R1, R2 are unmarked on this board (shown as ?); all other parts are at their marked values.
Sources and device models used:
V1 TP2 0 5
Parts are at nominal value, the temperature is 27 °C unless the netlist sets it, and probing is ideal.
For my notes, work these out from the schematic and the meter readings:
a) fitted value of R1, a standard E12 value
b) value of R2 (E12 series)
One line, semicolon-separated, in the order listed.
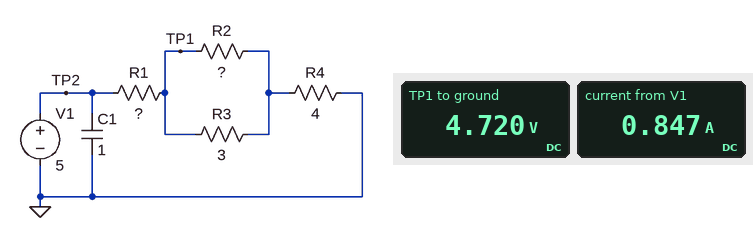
0.33 Ω; 3.3 Ω
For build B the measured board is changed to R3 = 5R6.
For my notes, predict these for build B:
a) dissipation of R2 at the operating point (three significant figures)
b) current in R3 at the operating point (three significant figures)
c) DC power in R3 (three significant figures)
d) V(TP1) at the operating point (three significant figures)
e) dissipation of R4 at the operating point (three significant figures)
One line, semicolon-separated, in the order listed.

796 mW; 289 mA; 469 mW; 4.74 V; 2.44 W
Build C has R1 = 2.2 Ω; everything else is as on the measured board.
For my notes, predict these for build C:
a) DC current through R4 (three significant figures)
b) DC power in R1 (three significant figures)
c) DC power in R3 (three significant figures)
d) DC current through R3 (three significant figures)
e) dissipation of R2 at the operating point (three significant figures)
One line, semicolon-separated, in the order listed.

643 mA; 911 mW; 341 mW; 337 mA; 310 mW
